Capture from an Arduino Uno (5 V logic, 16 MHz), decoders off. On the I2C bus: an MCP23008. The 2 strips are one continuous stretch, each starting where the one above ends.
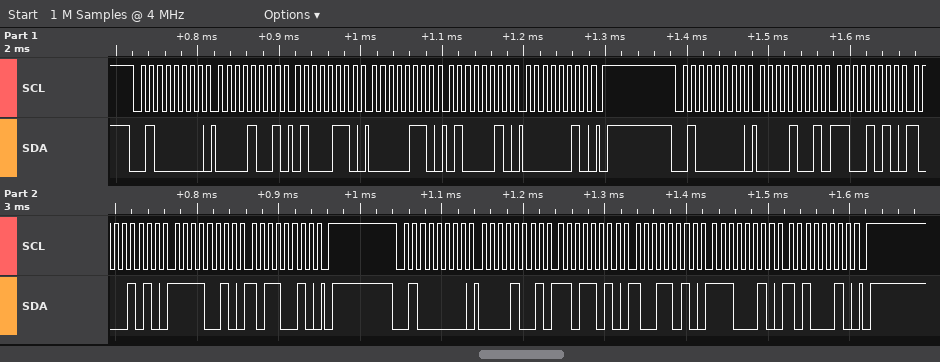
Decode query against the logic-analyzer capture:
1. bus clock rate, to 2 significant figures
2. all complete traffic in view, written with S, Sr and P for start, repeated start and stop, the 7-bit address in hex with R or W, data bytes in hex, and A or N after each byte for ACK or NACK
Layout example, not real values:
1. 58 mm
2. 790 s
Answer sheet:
1. 100 kHz
2. S 20W A 09 A 46 A 06 A 42 A 02 A P S 20W A 09 A CA A 8A A F2 A B2 A P S 20W A 09 A DA A 9A A E2 A A2 A P
